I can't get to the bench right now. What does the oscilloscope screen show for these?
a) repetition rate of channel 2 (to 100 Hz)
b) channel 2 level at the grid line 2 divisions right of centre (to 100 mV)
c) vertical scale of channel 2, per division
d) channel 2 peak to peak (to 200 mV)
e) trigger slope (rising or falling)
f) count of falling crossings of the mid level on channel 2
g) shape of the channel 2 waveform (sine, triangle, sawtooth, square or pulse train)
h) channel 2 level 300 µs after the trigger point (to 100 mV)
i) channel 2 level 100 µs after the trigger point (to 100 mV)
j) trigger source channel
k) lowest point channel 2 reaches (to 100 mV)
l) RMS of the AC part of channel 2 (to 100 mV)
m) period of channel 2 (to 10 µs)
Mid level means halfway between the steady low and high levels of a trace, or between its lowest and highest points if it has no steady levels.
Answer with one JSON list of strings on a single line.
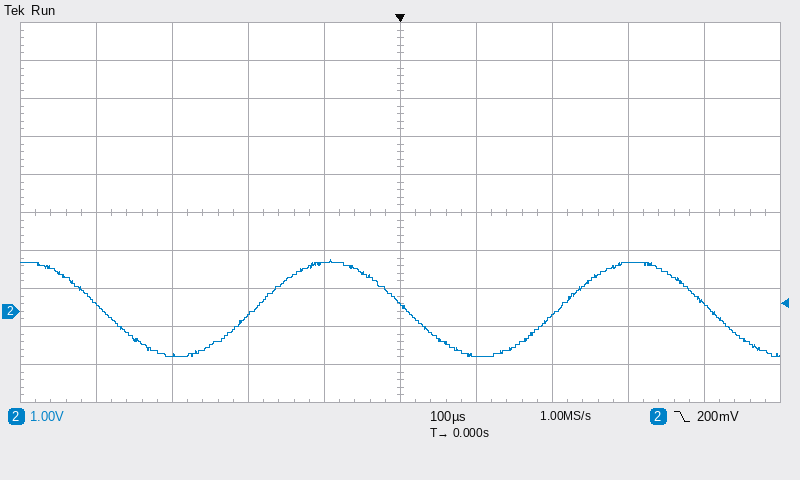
["2.5 kHz", "-100 mV", "1 V", "2.6 V", "falling", "3", "sine", "1.3 V", "-1.2 V", "channel 2", "-1.2 V", "900 mV", "400 µs"]
